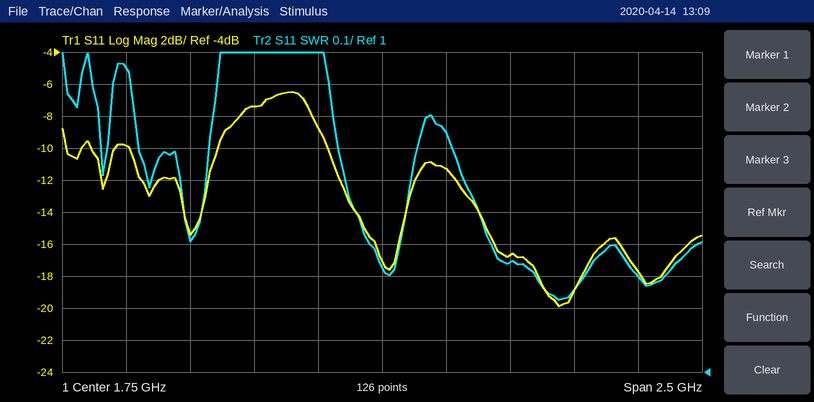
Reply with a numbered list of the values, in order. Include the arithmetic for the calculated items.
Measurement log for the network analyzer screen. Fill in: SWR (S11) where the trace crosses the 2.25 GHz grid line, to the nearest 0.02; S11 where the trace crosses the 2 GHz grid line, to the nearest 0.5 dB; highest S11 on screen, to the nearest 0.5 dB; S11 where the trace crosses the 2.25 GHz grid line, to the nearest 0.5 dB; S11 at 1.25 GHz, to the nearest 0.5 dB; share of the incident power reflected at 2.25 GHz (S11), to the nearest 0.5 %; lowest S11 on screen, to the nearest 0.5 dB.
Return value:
1. 1.34
2. -11.5 dB
3. -6.5 dB
4. -16.5 dB
5. -7.5 dB
6. 10^(-16.5/10) ≈ 2.24 %, so 2.0 % to the nearest 0.5 %
7. -20.0 dB
